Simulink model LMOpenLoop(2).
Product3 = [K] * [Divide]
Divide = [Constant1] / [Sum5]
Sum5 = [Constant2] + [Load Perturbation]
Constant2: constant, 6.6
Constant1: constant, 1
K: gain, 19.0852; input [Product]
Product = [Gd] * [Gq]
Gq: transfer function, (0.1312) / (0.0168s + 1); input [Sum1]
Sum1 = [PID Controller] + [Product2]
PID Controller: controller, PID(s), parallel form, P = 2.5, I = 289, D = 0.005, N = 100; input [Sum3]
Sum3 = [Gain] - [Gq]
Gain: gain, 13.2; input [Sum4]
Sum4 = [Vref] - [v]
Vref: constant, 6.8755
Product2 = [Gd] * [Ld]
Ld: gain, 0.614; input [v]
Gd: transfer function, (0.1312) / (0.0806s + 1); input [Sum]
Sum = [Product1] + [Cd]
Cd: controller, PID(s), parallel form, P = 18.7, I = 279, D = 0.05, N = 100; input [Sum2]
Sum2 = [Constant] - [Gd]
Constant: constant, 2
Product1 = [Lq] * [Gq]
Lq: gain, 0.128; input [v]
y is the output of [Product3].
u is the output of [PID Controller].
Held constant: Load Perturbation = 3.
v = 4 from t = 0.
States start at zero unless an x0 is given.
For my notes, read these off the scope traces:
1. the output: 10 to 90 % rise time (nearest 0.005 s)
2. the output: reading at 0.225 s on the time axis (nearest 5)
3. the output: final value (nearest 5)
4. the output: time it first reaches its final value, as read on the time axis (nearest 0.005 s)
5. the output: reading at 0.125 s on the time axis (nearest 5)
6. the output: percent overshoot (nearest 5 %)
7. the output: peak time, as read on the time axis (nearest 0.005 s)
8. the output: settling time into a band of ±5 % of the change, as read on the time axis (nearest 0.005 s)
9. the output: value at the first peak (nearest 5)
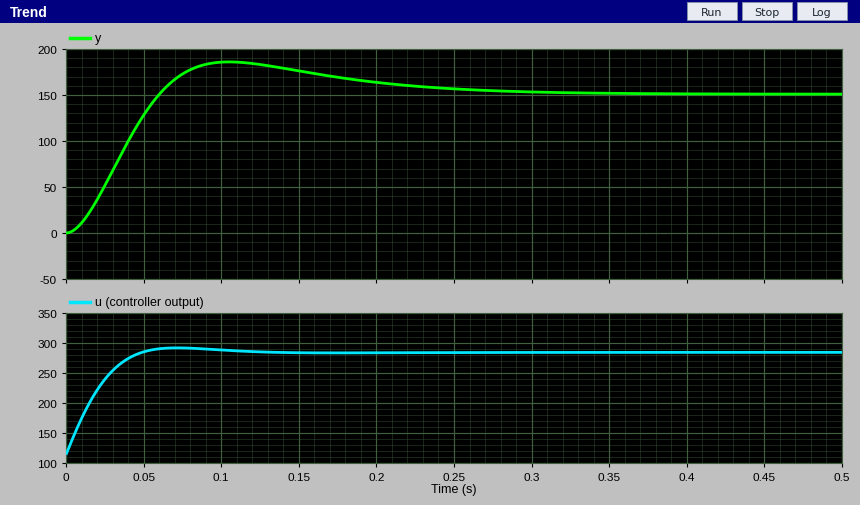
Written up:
0.040 s
160
150
0.060 s
185
25 %
0.105 s
0.235 s
185
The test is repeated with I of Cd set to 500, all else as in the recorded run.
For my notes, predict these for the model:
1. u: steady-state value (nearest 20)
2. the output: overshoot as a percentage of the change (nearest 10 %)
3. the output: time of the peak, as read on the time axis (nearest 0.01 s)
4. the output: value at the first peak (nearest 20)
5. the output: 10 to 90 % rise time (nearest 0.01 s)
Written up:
280
30 %
0.09 s
200
0.04 s
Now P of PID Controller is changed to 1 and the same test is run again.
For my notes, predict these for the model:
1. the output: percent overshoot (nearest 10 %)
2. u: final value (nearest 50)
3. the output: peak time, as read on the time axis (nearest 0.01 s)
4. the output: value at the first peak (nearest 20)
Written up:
30 %
300
0.10 s
200
